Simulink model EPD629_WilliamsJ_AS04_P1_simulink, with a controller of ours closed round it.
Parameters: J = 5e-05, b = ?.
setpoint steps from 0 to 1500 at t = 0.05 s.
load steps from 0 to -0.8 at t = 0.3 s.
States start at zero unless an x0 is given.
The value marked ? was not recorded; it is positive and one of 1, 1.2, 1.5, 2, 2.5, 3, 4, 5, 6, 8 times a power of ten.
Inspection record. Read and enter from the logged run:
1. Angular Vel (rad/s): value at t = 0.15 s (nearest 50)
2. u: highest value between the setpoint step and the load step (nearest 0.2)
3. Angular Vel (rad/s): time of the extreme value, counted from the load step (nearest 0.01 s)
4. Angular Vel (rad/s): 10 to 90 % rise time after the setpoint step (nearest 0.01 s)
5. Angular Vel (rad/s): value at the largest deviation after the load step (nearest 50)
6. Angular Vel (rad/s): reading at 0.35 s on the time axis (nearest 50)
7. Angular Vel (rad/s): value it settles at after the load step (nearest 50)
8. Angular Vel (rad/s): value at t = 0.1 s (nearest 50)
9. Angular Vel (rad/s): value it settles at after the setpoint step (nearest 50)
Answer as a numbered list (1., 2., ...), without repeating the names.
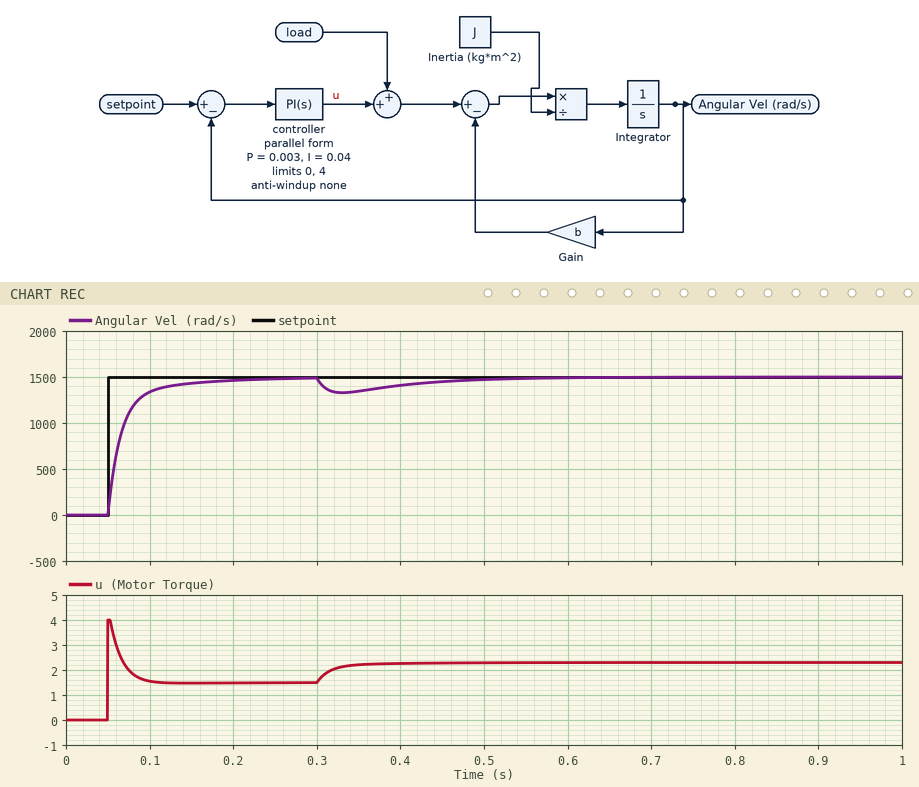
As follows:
1. 1450
2. 4.0
3. 0.03 s
4. 0.05 s
5. 1350
6. 1350
7. 1500
8. 1350
9. 1500
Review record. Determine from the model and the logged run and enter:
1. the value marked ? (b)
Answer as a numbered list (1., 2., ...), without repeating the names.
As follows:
1. 0.001
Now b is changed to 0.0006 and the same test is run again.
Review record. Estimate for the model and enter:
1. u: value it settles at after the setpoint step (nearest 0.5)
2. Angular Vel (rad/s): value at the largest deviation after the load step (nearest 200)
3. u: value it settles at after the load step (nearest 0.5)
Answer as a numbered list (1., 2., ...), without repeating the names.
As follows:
1. 1.0
2. 1400
3. 1.5
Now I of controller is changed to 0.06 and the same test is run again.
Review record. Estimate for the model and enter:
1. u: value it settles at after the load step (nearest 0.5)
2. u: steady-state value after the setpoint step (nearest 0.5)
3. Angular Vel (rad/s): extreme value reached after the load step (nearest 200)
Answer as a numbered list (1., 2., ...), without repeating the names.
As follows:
1. 2.5
2. 1.5
3. 1400
